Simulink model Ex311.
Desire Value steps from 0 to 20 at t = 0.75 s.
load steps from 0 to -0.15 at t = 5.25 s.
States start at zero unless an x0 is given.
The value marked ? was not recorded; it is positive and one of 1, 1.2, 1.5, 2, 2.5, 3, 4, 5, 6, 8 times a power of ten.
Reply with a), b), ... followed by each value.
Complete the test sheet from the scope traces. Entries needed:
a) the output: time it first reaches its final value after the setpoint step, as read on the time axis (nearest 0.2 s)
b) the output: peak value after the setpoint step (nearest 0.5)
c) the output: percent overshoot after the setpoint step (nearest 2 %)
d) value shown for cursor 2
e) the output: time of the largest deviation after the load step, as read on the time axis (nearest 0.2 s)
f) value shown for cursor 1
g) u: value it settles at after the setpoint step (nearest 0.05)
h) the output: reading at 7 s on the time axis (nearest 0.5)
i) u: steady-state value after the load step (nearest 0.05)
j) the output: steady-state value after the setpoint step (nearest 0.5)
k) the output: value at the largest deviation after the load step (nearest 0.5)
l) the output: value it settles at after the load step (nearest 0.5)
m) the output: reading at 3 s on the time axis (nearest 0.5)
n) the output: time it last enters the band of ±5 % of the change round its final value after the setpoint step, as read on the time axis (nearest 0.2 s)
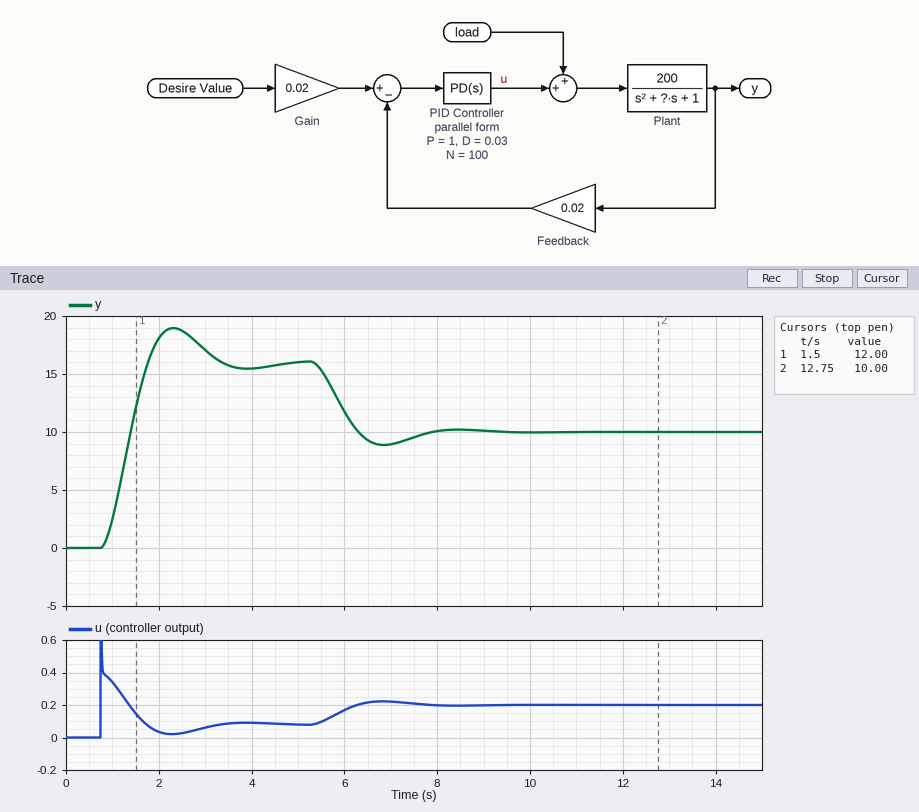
a) 1.8 s
b) 19.0
c) 18 %
d) 10.00
e) 6.8 s
f) 12.00
g) 0.10
h) 9.0
i) 0.20
j) 16.0
k) 9.0
l) 10.0
m) 17.0
n) 3.0 s
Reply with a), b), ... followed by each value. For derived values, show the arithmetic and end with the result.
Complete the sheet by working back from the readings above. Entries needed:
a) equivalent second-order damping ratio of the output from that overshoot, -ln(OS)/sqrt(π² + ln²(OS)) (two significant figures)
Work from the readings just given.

a) ln(0.18) = -1.715; 1.715 / sqrt(9.870 + 2.941) = 0.48
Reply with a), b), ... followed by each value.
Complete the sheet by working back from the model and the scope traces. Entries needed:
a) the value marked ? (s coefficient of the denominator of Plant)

a) 2
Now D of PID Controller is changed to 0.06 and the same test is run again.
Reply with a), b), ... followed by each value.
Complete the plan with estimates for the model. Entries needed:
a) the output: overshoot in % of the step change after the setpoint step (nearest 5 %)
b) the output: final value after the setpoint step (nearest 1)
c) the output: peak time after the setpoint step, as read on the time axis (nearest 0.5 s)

a) 15 %
b) 16
c) 2.5 s
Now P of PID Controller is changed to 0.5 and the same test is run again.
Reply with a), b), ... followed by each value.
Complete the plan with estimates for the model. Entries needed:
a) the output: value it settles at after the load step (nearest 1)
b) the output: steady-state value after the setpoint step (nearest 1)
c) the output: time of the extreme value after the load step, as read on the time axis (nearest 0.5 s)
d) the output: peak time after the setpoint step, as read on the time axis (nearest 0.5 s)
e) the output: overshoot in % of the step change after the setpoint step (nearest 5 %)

a) 3
b) 13
c) 7.5 s
d) 3.0 s
e) 10 %
